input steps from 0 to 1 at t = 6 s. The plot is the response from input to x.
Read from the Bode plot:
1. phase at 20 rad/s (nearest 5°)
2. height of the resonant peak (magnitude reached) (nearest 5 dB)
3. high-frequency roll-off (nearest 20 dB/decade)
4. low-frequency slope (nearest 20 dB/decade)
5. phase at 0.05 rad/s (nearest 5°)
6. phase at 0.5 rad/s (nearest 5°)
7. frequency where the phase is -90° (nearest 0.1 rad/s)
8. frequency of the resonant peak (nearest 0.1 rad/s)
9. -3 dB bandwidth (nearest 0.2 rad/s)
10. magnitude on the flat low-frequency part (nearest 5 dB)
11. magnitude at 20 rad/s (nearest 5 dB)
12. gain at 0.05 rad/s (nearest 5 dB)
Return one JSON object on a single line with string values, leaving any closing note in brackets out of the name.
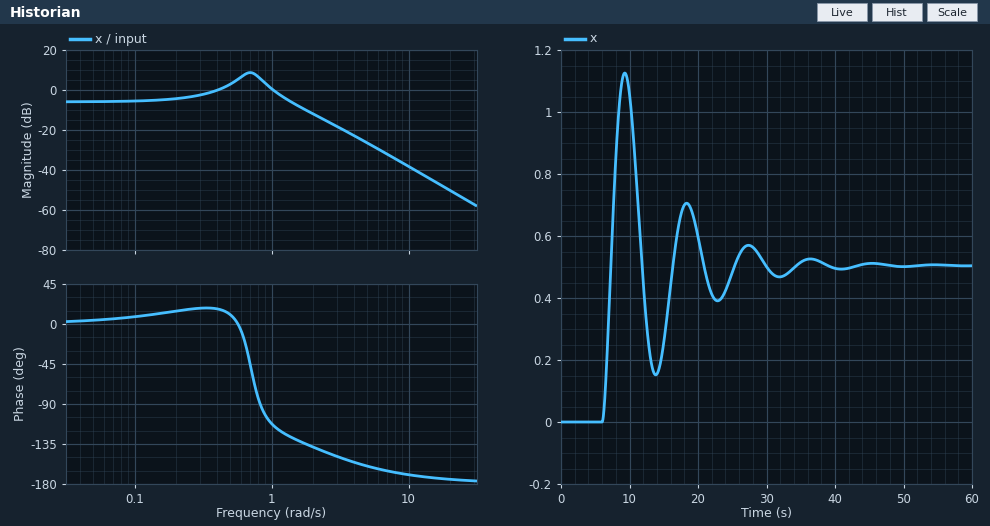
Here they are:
{"phase at 20 rad/s": "-175°", "height of the resonant peak (magnitude reached)": "10 dB", "high-frequency roll-off": "-40 dB/decade", "low-frequency slope": "0 dB/decade", "phase at 0.05 rad/s": "5°", "phase at 0.5 rad/s": "10°", "frequency where the phase is -90°": "0.8 rad/s", "frequency of the resonant peak": "0.7 rad/s", "-3 dB bandwidth": "1.6 rad/s", "magnitude on the flat low-frequency part": "-5 dB", "magnitude at 20 rad/s": "-50 dB", "gain at 0.05 rad/s": "-5 dB"}
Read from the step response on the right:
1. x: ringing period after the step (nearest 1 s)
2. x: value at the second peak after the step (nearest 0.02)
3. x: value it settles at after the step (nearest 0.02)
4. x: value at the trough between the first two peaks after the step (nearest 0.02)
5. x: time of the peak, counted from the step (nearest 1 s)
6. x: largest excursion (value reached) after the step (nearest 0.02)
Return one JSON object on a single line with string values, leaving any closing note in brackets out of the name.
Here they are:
{"x: ringing period after the step": "9 s", "x: value at the second peak after the step": "0.70", "x: value it settles at after the step": "0.50", "x: value at the trough between the first two peaks after the step": "0.16", "x: time of the peak, counted from the step": "3 s", "x: largest excursion (value reached) after the step": "1.12"}
